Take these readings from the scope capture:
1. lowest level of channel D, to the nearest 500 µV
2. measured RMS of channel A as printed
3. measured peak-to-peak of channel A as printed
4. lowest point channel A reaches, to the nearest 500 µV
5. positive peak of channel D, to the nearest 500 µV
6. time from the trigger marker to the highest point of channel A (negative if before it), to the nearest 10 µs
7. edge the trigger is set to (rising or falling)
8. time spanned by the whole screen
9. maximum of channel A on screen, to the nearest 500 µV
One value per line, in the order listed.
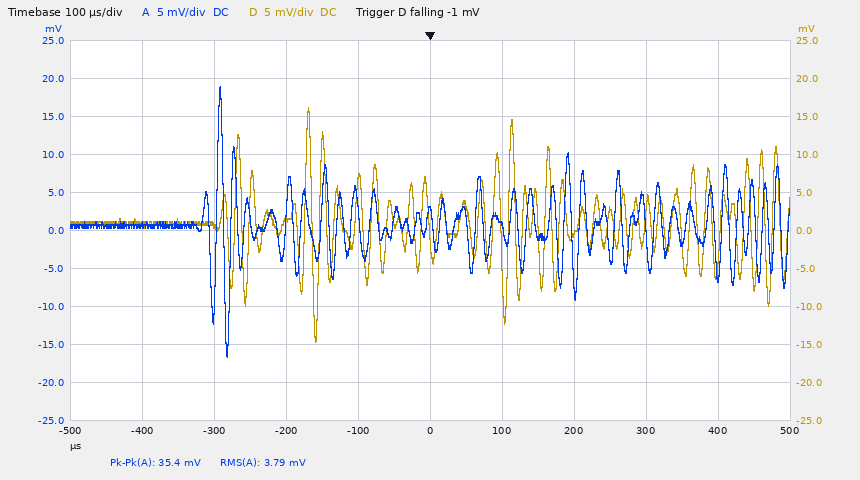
-14.5 mV
3.79 mV
35.4 mV
-16.5 mV
16.0 mV
-290 µs
falling
1 ms
19.0 mV
